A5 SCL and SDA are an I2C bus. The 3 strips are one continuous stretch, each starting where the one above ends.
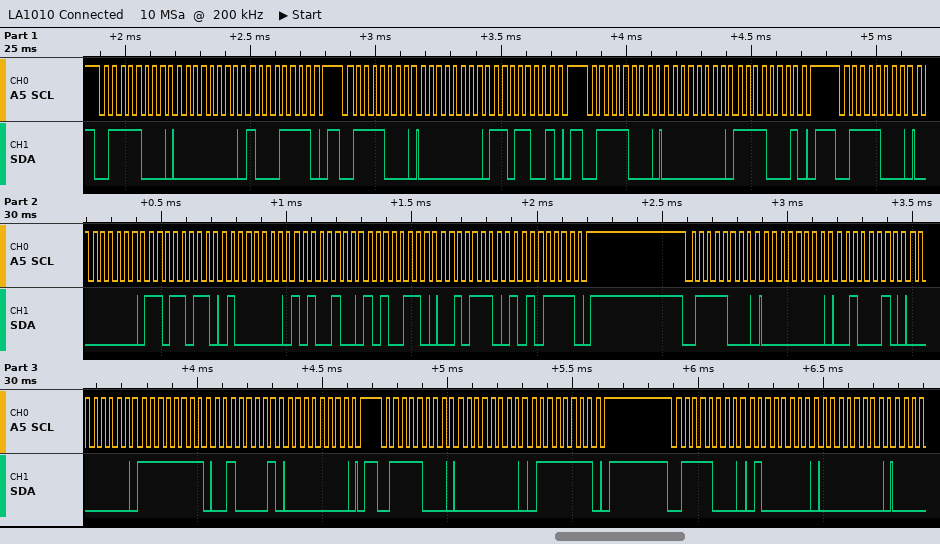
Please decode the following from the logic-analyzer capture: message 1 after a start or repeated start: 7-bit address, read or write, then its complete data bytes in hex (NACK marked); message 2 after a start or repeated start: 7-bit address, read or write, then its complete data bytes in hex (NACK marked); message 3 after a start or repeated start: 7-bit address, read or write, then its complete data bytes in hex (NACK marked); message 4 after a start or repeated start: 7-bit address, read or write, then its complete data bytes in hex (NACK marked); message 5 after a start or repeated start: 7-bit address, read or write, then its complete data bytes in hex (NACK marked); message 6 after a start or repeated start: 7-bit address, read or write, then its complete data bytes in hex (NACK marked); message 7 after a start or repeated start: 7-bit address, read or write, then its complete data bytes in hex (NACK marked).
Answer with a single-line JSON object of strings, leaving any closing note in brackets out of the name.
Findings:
{"message 1 after a start or repeated start: 7-bit address, read or write, then its complete data bytes in hex": "0x3C write: 00 8F", "message 2 after a start or repeated start: 7-bit address, read or write, then its complete data bytes in hex": "0x3C write: 00 D9", "message 3 after a start or repeated start: 7-bit address, read or write, then its complete data bytes in hex": "0x3C write: 00 F1", "message 4 after a start or repeated start: 7-bit address, read or write, then its complete data bytes in hex": "0x3C write: 00 DB 40 A4 A6 2E AF", "message 5 after a start or repeated start: 7-bit address, read or write, then its complete data bytes in hex": "0x3C write: 00 22 00 FF 21 00", "message 6 after a start or repeated start: 7-bit address, read or write, then its complete data bytes in hex": "0x3C write: 00 7F", "message 7 after a start or repeated start: 7-bit address, read or write, then its complete data bytes in hex": "0x3C write: 40 00"}
